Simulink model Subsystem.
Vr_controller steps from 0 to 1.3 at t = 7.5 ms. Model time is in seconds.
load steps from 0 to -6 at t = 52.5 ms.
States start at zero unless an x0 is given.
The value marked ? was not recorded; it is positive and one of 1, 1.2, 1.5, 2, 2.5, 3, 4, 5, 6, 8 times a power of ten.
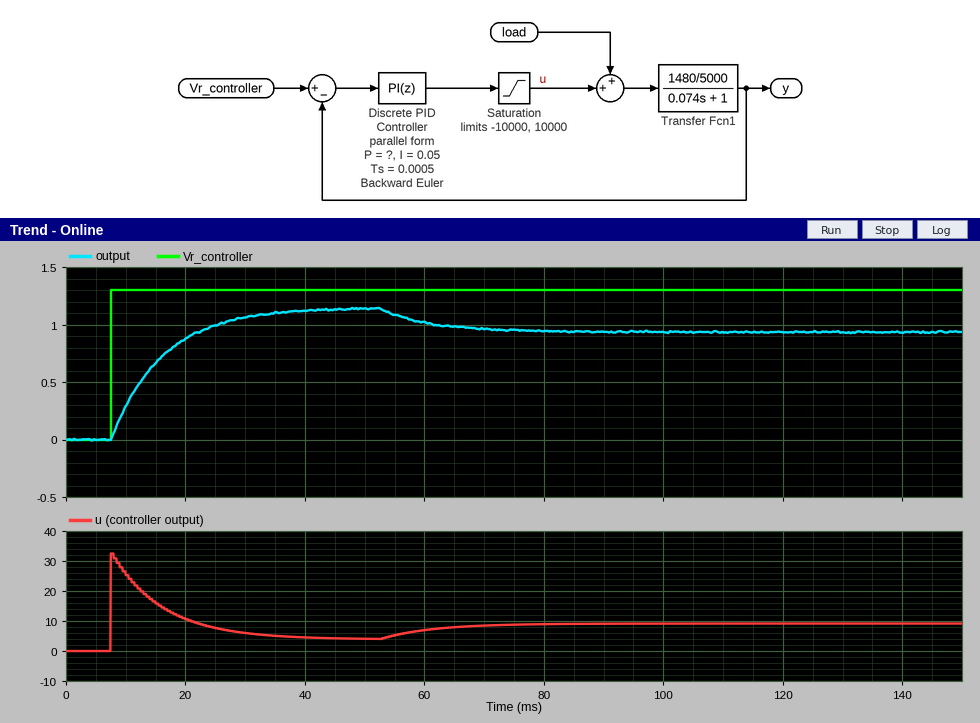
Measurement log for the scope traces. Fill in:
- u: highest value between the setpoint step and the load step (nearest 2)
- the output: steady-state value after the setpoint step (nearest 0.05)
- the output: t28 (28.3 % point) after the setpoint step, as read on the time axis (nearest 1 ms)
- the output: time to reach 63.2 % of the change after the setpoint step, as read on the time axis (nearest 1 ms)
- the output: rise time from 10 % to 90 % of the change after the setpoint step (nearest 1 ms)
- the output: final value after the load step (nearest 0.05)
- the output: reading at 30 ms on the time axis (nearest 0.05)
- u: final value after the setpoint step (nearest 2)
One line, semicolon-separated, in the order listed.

32; 1.15; 10 ms; 16 ms; 19 ms; 0.95; 1.05; 4
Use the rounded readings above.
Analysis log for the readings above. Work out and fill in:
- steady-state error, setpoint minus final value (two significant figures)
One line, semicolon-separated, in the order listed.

0.15
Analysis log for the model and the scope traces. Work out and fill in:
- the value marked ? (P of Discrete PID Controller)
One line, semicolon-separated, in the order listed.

25
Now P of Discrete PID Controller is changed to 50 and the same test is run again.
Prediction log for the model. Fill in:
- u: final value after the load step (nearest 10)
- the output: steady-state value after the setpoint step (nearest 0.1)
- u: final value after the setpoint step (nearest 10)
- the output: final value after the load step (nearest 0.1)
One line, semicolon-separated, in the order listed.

10; 1.2; 0; 1.1
